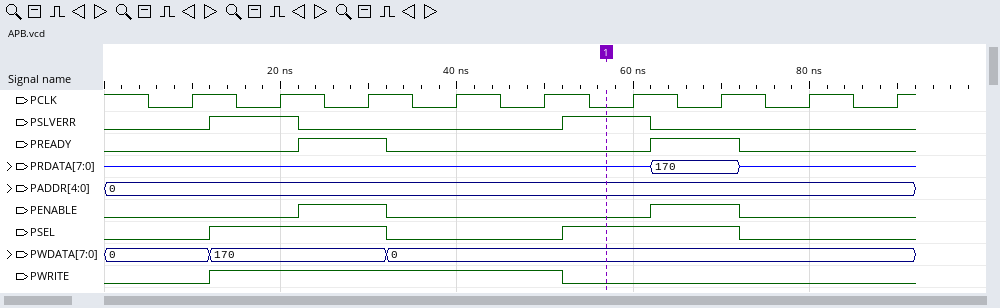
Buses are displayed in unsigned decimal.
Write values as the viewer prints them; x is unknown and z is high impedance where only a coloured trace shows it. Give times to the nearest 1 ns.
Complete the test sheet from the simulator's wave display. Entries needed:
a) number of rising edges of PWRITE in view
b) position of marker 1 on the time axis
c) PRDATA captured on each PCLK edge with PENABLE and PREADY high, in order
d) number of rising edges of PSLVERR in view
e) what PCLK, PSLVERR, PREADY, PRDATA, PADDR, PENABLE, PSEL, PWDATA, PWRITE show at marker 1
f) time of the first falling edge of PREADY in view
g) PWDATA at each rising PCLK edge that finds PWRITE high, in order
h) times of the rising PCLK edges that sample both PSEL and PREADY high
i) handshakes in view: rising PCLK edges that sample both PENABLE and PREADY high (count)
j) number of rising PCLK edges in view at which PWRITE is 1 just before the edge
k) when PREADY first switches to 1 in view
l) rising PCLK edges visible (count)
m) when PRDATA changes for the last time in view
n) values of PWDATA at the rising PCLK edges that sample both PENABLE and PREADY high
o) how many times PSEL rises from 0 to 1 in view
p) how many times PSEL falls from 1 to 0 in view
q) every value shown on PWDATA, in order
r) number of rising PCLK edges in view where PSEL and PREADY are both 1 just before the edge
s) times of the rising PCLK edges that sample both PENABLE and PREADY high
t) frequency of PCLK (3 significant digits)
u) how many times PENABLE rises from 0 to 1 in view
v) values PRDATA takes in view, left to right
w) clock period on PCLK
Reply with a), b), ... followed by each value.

a) 1
b) 57 ns
c) z, 170
d) 2
e) PCLK=0, PSLVERR=1, PREADY=0, PRDATA=z, PADDR=0, PENABLE=0, PSEL=1, PWDATA=0, PWRITE=0
f) 32 ns
g) 170, 170, 0, 0
h) 30 ns, 70 ns
i) 2
j) 4
k) 22 ns
l) 9
m) 72 ns
n) 170, 0
o) 2
p) 2
q) 0, 170, 0
r) 2
s) 30 ns, 70 ns
t) 100 MHz
u) 2
v) z, 170, z
w) 10 ns
